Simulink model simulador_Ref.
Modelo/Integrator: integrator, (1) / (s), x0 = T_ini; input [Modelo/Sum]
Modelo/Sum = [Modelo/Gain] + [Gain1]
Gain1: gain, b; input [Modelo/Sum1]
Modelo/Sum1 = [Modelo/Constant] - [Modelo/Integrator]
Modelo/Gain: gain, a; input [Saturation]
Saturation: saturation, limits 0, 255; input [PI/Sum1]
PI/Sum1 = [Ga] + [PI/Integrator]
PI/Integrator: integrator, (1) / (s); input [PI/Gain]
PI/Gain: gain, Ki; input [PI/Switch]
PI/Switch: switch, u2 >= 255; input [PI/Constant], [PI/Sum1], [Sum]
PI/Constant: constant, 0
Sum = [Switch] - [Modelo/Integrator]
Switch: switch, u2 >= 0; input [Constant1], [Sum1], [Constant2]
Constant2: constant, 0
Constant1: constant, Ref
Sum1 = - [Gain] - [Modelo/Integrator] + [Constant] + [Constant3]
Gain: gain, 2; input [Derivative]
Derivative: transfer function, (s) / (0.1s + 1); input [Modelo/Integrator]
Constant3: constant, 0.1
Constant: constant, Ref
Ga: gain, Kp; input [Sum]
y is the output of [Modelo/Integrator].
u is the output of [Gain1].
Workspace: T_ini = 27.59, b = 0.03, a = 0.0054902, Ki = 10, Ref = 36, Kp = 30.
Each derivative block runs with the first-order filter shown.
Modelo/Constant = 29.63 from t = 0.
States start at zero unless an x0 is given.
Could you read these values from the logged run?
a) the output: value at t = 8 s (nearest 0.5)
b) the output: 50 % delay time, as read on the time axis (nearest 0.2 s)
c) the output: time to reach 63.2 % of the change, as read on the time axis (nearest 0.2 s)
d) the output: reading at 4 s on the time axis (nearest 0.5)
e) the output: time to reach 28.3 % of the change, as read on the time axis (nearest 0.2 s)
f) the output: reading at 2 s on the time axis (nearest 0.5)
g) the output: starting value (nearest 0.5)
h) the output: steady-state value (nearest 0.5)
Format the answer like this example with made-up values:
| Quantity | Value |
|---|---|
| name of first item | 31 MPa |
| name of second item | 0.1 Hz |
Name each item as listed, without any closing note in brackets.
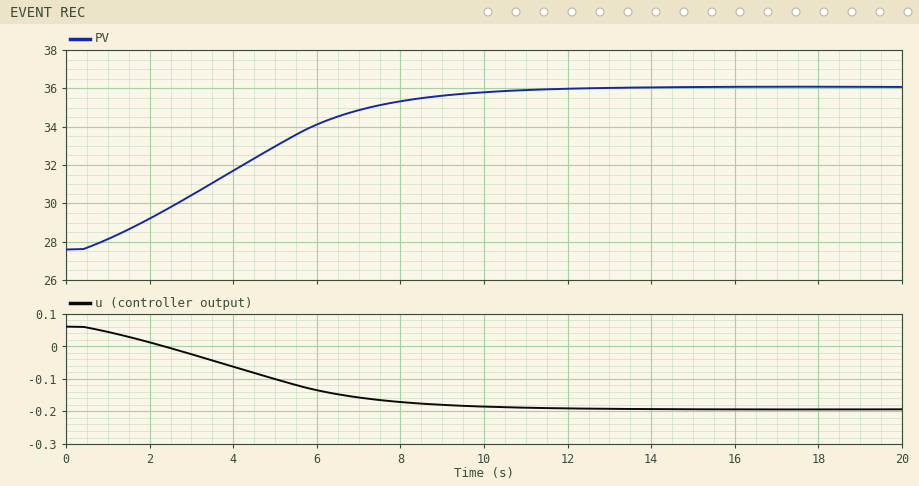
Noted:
| Quantity | Value |
|---|---|
| the output: value at t = 8 s | 35.5 |
| the output: 50 % delay time, as read on the time axis | 4.0 s |
| the output: time to reach 63.2 % of the change, as read on the time axis | 5.0 s |
| the output: reading at 4 s on the time axis | 31.5 |
| the output: time to reach 28.3 % of the change, as read on the time axis | 2.6 s |
| the output: reading at 2 s on the time axis | 29.0 |
| the output: starting value | 27.5 |
| the output: steady-state value | 36.0 |
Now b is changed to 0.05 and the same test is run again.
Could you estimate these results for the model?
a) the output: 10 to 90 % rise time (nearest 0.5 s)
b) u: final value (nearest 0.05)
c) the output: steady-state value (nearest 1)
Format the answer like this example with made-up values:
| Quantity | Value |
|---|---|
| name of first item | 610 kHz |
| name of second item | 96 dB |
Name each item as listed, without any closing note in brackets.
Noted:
| Quantity | Value |
|---|---|
| the output: 10 to 90 % rise time | 6.5 s |
| u: final value | -0.30 |
| the output: steady-state value | 36 |
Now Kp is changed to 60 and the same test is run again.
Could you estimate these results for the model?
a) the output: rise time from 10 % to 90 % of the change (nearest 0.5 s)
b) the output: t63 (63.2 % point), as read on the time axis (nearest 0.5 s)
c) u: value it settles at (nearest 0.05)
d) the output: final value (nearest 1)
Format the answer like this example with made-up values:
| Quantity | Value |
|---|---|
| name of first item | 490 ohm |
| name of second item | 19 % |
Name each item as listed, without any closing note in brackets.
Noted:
| Quantity | Value |
|---|---|
| the output: rise time from 10 % to 90 % of the change | 7.0 s |
| the output: t63 (63.2 % point), as read on the time axis | 4.5 s |
| u: value it settles at | -0.20 |
| the output: final value | 36 |
